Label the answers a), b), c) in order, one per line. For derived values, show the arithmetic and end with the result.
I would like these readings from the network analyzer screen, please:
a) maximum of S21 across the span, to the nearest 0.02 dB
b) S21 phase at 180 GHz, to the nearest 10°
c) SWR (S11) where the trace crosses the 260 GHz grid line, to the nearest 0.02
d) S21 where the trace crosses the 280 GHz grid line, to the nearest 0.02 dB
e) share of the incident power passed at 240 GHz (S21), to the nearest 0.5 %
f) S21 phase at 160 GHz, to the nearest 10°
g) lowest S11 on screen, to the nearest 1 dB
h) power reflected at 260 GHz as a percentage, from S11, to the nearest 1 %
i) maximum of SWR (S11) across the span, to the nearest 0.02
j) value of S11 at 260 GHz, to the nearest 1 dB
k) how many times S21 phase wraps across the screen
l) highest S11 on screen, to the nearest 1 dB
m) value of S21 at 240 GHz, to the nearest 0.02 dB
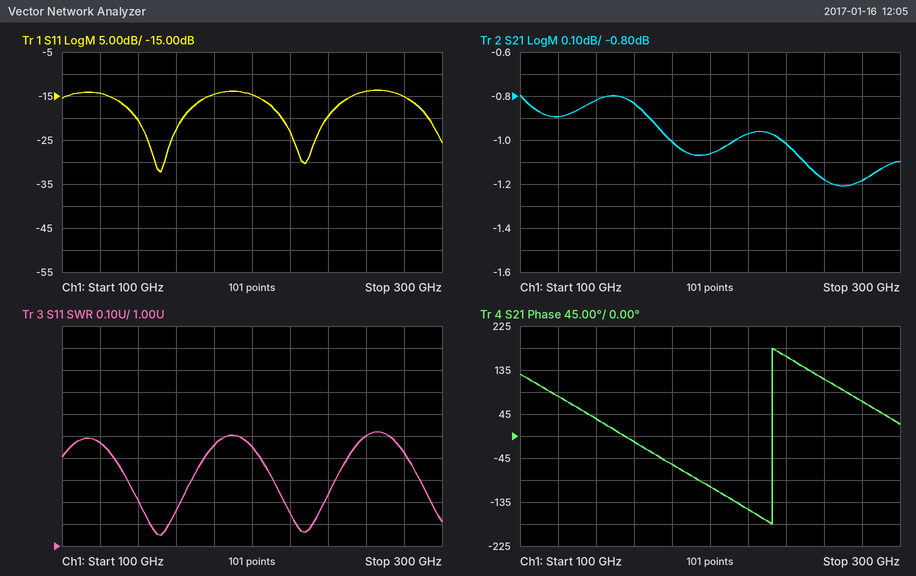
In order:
a) -0.80 dB
b) -60°
c) 1.50
d) -1.18 dB
e) 10^(-1.02/10) ≈ 79.1 %, so 79.0 % to the nearest 0.5 %
f) -10°
g) -32 dB
h) 10^(-14/10) ≈ 4 %
i) 1.52
j) -14 dB
k) 1
l) -14 dB
m) -1.02 dB
